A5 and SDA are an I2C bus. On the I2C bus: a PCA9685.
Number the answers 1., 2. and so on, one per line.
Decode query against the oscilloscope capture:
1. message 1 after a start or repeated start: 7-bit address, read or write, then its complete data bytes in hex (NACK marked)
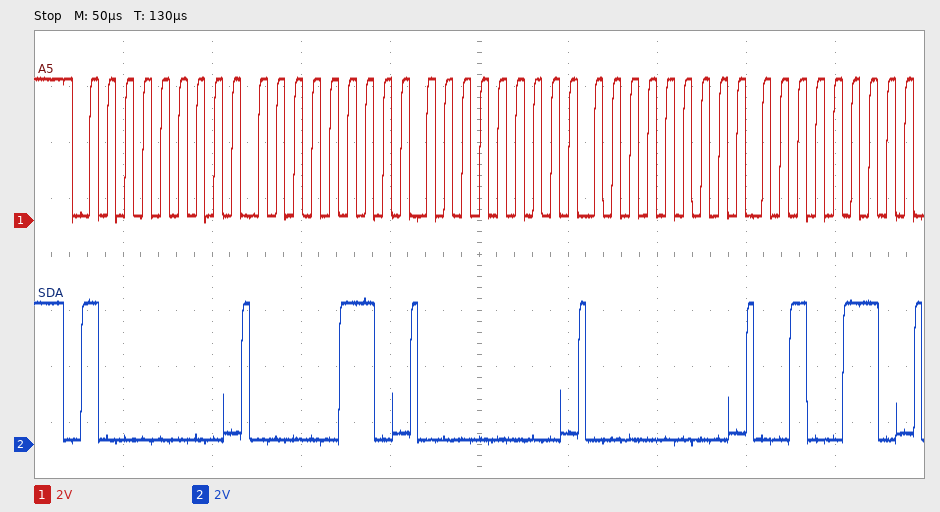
1. 0x40 write: 06 00 00 26
